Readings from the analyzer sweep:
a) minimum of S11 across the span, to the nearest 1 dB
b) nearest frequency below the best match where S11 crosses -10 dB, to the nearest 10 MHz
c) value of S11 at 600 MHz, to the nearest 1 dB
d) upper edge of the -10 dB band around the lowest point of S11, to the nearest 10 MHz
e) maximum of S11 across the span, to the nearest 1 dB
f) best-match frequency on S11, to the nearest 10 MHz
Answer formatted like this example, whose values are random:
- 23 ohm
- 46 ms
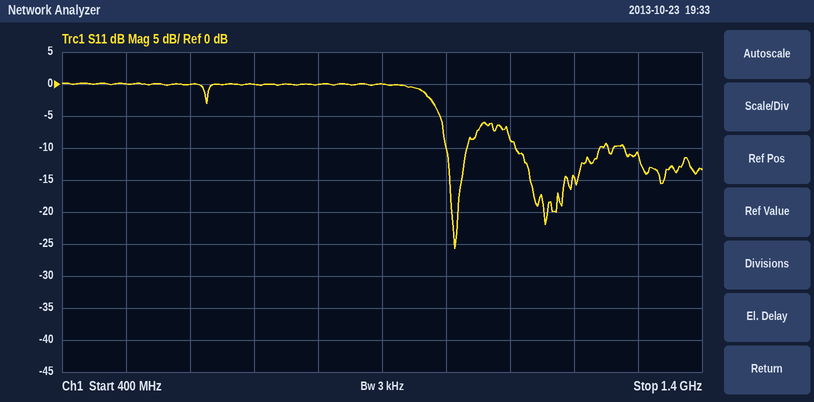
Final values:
- -26 dB
- 1.00 GHz
- 0 dB
- 1.03 GHz
- 0 dB
- 1.01 GHz
